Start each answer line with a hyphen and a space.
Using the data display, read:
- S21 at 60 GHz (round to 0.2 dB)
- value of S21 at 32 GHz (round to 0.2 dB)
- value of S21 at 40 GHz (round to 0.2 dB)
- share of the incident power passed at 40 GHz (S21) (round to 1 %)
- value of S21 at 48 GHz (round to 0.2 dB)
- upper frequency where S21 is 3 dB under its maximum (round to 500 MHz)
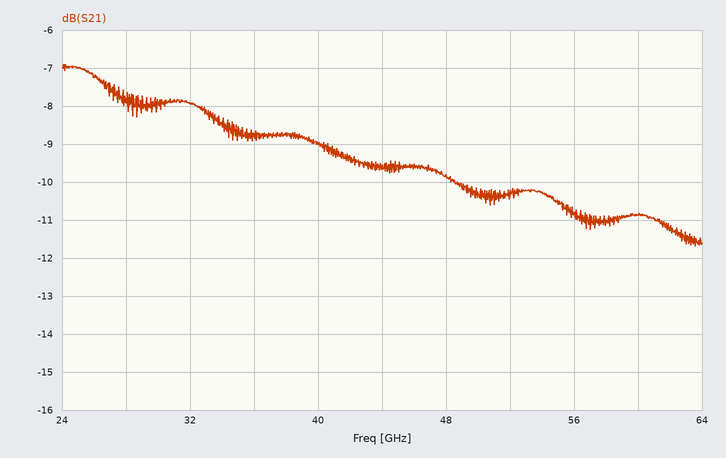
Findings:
- -10.8 dB
- -8.0 dB
- -9.0 dB
- 13 %
- -9.8 dB
- 48.0 GHz
